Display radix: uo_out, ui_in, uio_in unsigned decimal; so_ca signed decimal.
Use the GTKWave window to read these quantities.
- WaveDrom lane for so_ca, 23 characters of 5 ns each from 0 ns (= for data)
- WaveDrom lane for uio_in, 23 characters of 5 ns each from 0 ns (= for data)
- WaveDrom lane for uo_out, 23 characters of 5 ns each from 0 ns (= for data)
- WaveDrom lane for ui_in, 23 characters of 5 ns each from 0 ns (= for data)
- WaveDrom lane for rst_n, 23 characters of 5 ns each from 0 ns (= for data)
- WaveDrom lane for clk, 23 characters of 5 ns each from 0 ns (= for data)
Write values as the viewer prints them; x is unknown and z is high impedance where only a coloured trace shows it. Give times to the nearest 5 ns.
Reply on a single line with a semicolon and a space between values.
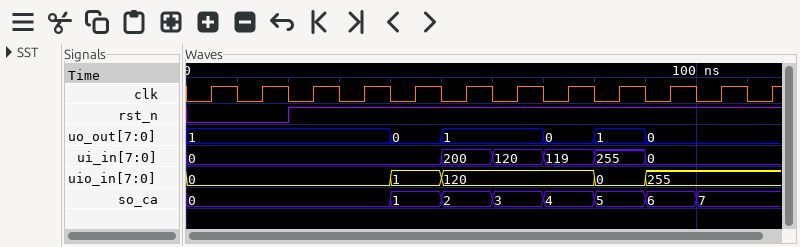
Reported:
{name: 'so_ca', wave: '=.......=.=.=.=.=.=.=..', data: '0 1 2 3 4 5 6 7'}; {name: 'uio_in', wave: '=.......=.=.....=.=....', data: '0 1 120 0 255'}; {name: 'uo_out', wave: '=.......=.=...=.=.=....', data: '1 0 1 0 1 0'}; {name: 'ui_in', wave: '=.........=.=.=.=.=....', data: '0 200 120 119 255 0'}; {name: 'rst_n', wave: '0...1..................'}; {name: 'clk', wave: '01010101010101010101010'}
